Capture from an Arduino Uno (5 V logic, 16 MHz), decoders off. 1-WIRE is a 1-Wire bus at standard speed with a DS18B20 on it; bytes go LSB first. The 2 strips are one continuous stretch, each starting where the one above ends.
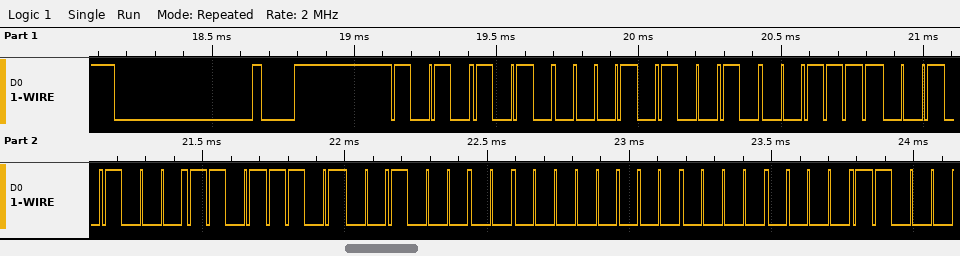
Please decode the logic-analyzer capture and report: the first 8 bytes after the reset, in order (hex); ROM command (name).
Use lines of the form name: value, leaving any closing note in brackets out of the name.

the first 8 bytes after the reset, in order: 55 28 F1 14 BB 04 00 00
ROM command: Match ROM
